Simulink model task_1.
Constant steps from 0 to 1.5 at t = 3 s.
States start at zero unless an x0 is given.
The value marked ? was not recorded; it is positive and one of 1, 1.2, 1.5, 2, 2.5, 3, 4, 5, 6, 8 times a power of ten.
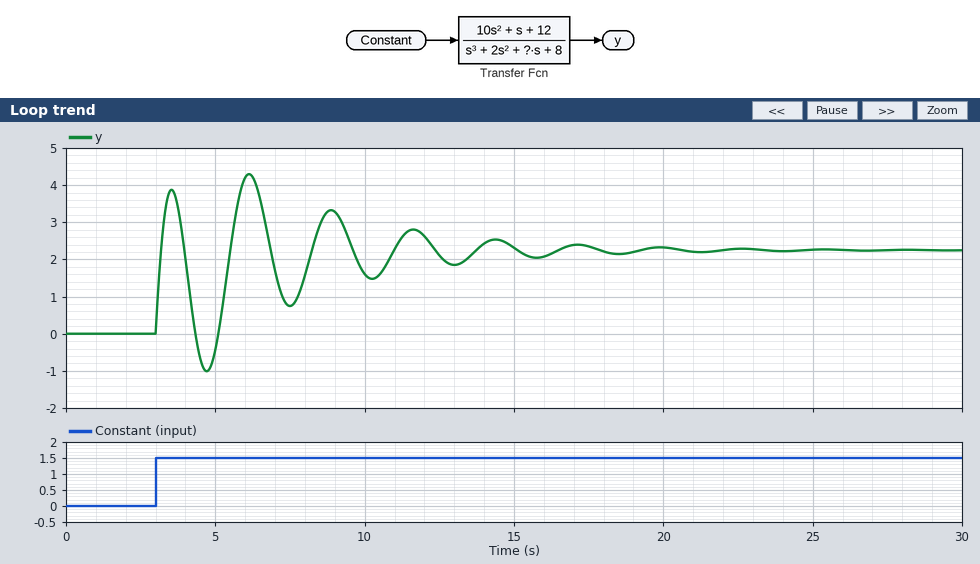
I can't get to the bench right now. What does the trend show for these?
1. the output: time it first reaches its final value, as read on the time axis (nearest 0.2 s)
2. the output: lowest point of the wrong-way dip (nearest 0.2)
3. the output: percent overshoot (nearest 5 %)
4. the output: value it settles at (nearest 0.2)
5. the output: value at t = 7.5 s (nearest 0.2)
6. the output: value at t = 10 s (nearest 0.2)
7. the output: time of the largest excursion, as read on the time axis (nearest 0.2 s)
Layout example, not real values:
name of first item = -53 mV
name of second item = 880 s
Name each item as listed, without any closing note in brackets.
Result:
the output: time it first reaches its final value, as read on the time axis = 3.2 s
the output: lowest point of the wrong-way dip = -1.0
the output: percent overshoot = 90 %
the output: value it settles at = 2.2
the output: value at t = 7.5 s = 0.8
the output: value at t = 10 s = 1.6
the output: time of the largest excursion, as read on the time axis = 6.2 s
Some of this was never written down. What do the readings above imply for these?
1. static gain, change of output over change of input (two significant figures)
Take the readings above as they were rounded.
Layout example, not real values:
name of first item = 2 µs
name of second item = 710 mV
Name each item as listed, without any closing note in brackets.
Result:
static gain, change of output over change of input = 1.5
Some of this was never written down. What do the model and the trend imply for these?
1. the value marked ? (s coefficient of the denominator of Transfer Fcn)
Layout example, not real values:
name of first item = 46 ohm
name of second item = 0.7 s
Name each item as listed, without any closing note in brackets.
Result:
the value marked ? = 6
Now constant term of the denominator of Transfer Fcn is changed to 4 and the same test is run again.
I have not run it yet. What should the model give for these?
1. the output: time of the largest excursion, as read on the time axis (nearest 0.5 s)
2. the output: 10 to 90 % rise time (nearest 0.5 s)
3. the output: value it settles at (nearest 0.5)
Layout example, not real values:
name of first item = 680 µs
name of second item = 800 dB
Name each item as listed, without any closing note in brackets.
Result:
the output: time of the largest excursion, as read on the time axis = 6.5 s
the output: 10 to 90 % rise time = 3.0 s
the output: value it settles at = 4.5
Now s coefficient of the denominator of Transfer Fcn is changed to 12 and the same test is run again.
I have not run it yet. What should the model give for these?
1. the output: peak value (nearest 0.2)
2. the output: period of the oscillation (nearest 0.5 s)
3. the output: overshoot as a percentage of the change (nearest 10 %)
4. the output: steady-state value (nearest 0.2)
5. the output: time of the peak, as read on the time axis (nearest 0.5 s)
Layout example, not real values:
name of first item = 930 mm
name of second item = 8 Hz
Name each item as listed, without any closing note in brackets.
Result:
the output: peak value = 3.0
the output: period of the oscillation = 2.0 s
the output: overshoot as a percentage of the change = 40 %
the output: steady-state value = 2.2
the output: time of the peak, as read on the time axis = 3.5 s
